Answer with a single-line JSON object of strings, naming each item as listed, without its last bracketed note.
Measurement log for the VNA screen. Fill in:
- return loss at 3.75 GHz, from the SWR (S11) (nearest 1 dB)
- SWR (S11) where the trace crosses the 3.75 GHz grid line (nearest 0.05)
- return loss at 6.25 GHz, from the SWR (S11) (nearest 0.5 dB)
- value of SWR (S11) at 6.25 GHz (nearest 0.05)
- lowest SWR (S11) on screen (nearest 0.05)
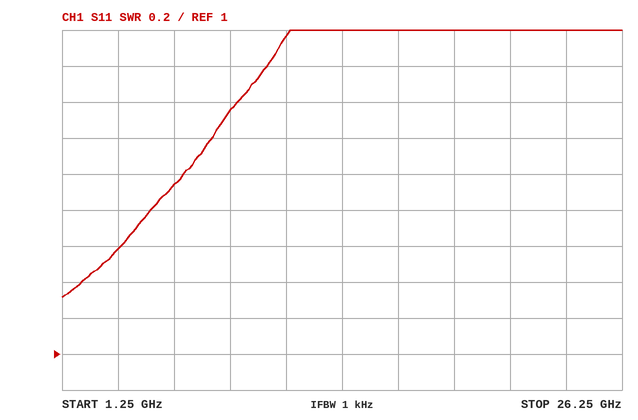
{"return loss at 3.75 GHz, from the SWR (S11)": "13 dB", "SWR (S11) where the trace crosses the 3.75 GHz grid line": "1.60", "return loss at 6.25 GHz, from the SWR (S11)": "10.0 dB", "value of SWR (S11) at 6.25 GHz": "1.95", "lowest SWR (S11) on screen": "1.30"}
